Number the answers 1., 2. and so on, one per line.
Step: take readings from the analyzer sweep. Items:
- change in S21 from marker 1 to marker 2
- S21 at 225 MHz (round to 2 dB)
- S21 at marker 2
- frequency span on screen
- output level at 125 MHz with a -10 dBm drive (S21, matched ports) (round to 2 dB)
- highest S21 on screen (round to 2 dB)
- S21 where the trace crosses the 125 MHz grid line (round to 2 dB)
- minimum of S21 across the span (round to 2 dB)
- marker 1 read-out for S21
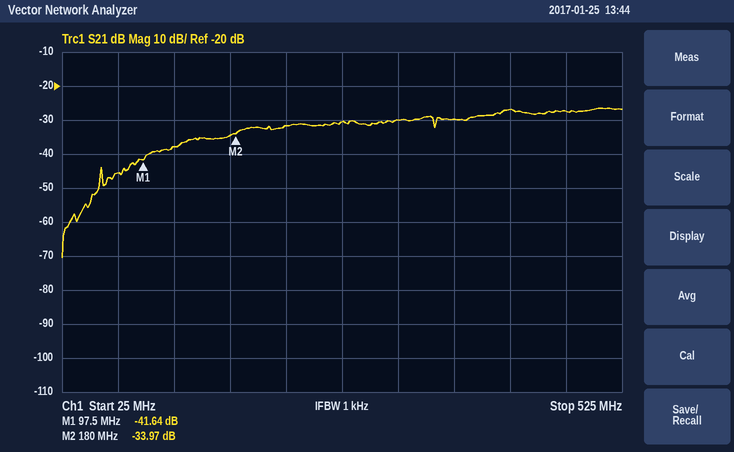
1. 7.67 dB
2. -32 dB
3. -33.97 dB
4. 500 MHz
5. -48 dBm
6. -26 dB
7. -38 dB
8. -70 dB
9. -41.64 dB
